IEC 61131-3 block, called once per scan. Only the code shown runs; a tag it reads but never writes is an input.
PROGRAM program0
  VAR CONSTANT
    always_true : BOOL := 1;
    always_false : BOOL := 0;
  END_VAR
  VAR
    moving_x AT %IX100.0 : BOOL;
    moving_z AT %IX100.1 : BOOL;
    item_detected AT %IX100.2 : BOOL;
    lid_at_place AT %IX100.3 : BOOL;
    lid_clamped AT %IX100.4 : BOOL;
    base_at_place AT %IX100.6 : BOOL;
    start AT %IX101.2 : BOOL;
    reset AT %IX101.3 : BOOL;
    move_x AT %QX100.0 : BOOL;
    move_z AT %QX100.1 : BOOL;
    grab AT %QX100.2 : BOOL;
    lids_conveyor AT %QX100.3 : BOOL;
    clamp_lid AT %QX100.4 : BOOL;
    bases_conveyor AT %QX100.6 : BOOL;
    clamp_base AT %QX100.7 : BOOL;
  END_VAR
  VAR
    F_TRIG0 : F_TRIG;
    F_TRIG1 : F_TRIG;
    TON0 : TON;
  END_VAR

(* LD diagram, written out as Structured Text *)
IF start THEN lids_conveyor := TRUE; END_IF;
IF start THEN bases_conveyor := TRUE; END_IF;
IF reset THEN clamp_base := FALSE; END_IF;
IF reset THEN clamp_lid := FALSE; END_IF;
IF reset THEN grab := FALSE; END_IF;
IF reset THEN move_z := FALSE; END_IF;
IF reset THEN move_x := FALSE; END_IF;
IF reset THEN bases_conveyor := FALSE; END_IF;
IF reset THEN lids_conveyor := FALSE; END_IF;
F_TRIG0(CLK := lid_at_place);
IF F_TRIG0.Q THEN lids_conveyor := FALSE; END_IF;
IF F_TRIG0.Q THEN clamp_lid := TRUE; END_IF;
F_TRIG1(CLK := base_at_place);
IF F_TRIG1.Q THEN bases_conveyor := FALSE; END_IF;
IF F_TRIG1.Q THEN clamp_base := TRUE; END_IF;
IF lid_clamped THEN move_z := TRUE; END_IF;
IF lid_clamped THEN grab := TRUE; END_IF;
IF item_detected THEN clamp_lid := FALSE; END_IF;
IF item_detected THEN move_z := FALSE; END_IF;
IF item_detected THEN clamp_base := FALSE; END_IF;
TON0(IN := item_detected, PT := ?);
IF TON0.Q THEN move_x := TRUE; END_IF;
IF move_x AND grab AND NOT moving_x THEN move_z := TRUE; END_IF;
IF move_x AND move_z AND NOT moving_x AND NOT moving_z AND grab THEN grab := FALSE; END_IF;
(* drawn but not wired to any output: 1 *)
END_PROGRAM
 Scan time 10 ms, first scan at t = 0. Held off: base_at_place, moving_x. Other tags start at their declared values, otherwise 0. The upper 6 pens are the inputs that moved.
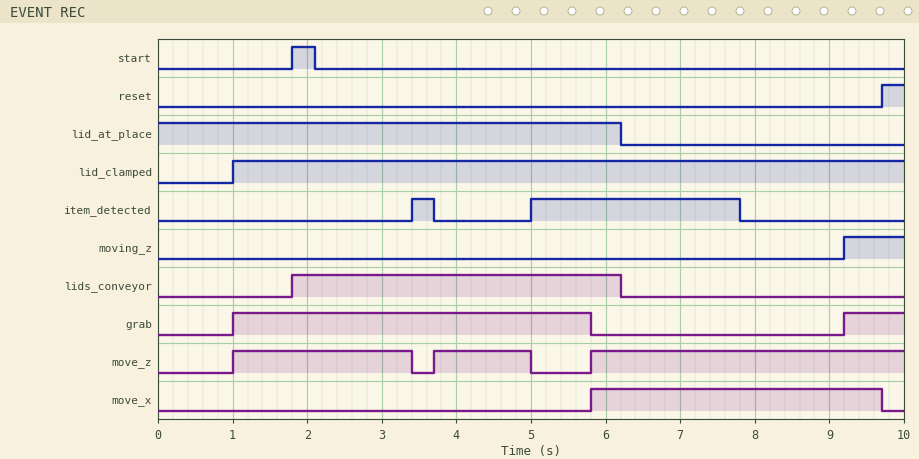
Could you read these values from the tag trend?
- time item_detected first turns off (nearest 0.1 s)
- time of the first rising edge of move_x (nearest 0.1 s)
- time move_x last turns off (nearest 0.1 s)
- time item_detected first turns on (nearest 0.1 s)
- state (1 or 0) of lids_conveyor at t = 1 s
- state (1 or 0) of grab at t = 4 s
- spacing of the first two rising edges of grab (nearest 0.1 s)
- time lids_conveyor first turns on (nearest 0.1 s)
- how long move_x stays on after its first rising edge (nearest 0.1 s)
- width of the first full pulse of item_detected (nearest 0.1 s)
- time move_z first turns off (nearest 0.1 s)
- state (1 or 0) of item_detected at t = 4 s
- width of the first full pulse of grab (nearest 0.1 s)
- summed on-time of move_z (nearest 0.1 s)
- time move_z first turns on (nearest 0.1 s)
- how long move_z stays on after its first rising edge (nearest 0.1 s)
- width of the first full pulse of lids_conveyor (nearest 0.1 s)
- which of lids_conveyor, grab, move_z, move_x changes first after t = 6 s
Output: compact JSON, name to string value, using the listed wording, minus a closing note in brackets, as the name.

{"time item_detected first turns off": "3.7 s", "time of the first rising edge of move_x": "5.8 s", "time move_x last turns off": "9.7 s", "time item_detected first turns on": "3.4 s", "state (1 or 0) of lids_conveyor at t = 1 s": "0", "state (1 or 0) of grab at t = 4 s": "1", "spacing of the first two rising edges of grab": "8.2 s", "time lids_conveyor first turns on": "1.8 s", "how long move_x stays on after its first rising edge": "3.9 s", "width of the first full pulse of item_detected": "0.3 s", "time move_z first turns off": "3.4 s", "state (1 or 0) of item_detected at t = 4 s": "0", "width of the first full pulse of grab": "4.8 s", "summed on-time of move_z": "7.9 s", "time move_z first turns on": "1.0 s", "how long move_z stays on after its first rising edge": "2.4 s", "width of the first full pulse of lids_conveyor": "4.4 s", "which of lids_conveyor, grab, move_z, move_x changes first after t = 6 s": "lids_conveyor"}
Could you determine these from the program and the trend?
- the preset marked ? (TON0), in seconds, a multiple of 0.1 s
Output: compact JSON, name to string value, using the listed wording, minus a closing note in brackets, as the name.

{"the preset marked ? (TON0), in seconds, a multiple of 0.1 s": "0.8 s"}
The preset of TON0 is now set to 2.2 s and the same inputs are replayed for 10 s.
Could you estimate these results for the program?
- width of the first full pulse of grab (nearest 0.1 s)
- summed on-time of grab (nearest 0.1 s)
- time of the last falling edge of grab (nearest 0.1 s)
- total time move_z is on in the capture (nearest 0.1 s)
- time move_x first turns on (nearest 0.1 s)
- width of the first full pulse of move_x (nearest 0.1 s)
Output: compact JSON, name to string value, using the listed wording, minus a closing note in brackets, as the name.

{"width of the first full pulse of grab": "6.2 s", "summed on-time of grab": "7.0 s", "time of the last falling edge of grab": "7.2 s", "total time move_z is on in the capture": "6.5 s", "time move_x first turns on": "7.2 s", "width of the first full pulse of move_x": "2.5 s"}
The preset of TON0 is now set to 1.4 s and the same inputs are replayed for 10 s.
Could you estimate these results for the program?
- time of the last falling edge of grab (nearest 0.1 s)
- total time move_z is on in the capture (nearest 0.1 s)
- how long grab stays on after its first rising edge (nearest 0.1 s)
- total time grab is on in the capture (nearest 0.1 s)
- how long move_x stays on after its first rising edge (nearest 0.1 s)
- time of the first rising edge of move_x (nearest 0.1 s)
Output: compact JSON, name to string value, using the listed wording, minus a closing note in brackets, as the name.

{"time of the last falling edge of grab": "6.4 s", "total time move_z is on in the capture": "7.3 s", "how long grab stays on after its first rising edge": "5.4 s", "total time grab is on in the capture": "6.2 s", "how long move_x stays on after its first rising edge": "3.3 s", "time of the first rising edge of move_x": "6.4 s"}
